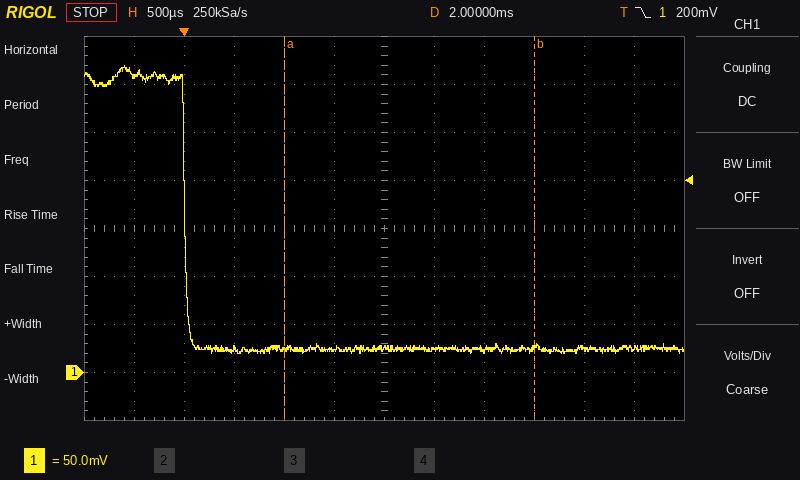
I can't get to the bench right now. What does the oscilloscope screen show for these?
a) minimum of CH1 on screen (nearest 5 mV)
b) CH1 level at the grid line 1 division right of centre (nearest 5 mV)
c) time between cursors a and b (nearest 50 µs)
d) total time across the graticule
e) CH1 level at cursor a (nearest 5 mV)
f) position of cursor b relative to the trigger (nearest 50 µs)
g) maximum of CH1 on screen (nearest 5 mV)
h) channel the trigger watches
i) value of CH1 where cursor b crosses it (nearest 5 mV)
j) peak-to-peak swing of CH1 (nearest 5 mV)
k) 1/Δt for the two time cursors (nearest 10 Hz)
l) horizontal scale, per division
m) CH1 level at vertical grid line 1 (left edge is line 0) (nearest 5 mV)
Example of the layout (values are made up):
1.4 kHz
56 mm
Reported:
20 mV
25 mV
2.50 ms
6 ms
25 mV
+3.50 ms
320 mV
CH1
25 mV
300 mV
400 Hz
500 µs
310 mV
